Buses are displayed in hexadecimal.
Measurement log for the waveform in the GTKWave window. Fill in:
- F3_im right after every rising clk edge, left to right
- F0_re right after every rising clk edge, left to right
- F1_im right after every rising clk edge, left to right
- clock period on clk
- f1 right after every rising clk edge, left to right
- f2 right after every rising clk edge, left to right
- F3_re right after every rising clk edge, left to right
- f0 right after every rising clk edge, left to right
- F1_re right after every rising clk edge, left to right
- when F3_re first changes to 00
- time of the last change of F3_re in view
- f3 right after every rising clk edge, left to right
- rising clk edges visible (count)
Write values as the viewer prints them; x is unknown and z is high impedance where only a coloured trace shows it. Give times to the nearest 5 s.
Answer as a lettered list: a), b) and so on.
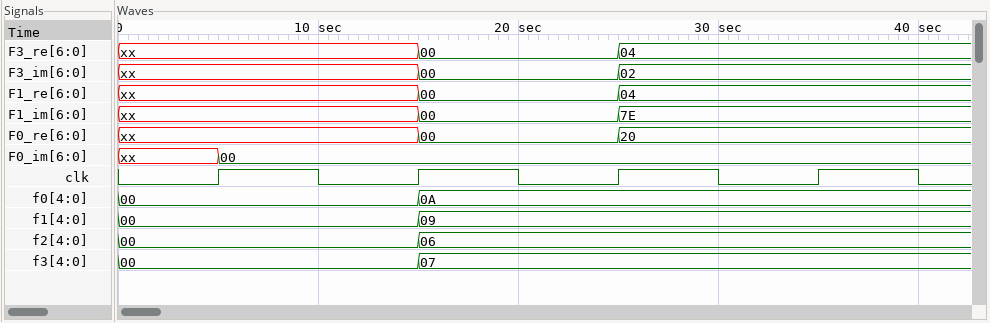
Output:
a) xx, 00, 02, 02
b) xx, 00, 20, 20
c) xx, 00, 7E, 7E
d) 10 s
e) 00, 09, 09, 09
f) 00, 06, 06, 06
g) xx, 00, 04, 04
h) 00, 0A, 0A, 0A
i) xx, 00, 04, 04
j) 15 s
k) 25 s
l) 00, 07, 07, 07
m) 4
